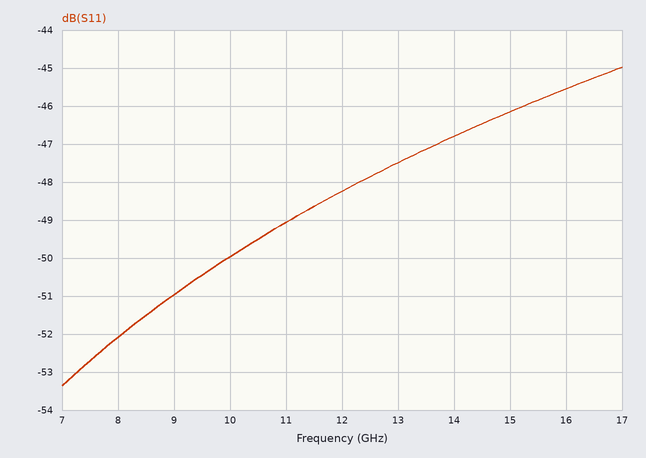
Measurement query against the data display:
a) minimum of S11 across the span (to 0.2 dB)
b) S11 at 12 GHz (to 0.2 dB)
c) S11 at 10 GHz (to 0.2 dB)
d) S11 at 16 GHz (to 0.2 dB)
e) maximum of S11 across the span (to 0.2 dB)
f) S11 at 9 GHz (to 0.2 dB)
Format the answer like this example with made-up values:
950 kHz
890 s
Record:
-53.4 dB
-48.2 dB
-50.0 dB
-45.6 dB
-45.0 dB
-51.0 dB
